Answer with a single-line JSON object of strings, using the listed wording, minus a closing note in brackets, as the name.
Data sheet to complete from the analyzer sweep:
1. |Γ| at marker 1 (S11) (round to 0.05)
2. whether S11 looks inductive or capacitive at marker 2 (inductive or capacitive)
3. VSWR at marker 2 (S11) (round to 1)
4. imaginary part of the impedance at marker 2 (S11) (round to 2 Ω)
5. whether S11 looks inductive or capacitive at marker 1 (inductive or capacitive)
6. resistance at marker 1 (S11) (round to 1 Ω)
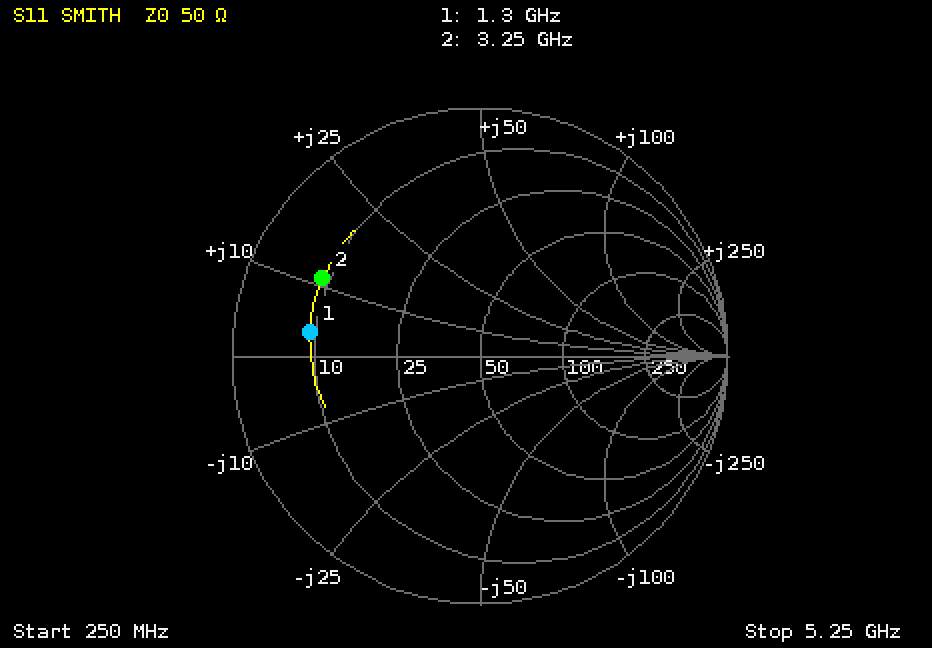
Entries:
{"|Γ| at marker 1 (S11)": "0.70", "whether S11 looks inductive or capacitive at marker 2": "inductive", "VSWR at marker 2 (S11)": "6", "imaginary part of the impedance at marker 2 (S11)": "+12 Ω", "whether S11 looks inductive or capacitive at marker 1": "inductive", "resistance at marker 1 (S11)": "9 Ω"}
